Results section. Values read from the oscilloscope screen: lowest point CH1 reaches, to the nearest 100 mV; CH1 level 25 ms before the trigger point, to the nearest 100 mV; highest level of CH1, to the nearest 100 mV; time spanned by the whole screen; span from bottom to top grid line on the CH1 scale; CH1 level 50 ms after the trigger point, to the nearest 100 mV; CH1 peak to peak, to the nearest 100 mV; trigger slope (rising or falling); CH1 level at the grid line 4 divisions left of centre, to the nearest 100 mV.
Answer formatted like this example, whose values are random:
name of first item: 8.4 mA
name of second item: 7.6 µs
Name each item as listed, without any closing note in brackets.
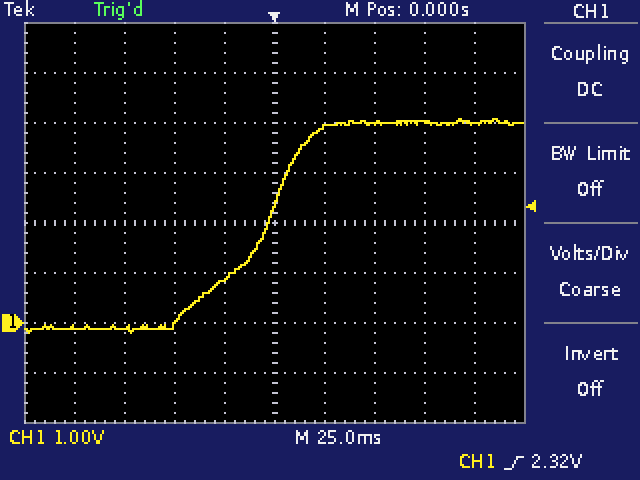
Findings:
lowest point CH1 reaches, to the nearest 100 mV: -200 mV
CH1 level 25 ms before the trigger point, to the nearest 100 mV: 900 mV
highest level of CH1, to the nearest 100 mV: 4.1 V
time spanned by the whole screen: 250 ms
span from bottom to top grid line on the CH1 scale: 8 V
CH1 level 50 ms after the trigger point, to the nearest 100 mV: 4.0 V
CH1 peak to peak, to the nearest 100 mV: 4.3 V
trigger slope: rising
CH1 level at the grid line 4 divisions left of centre, to the nearest 100 mV: -100 mV
